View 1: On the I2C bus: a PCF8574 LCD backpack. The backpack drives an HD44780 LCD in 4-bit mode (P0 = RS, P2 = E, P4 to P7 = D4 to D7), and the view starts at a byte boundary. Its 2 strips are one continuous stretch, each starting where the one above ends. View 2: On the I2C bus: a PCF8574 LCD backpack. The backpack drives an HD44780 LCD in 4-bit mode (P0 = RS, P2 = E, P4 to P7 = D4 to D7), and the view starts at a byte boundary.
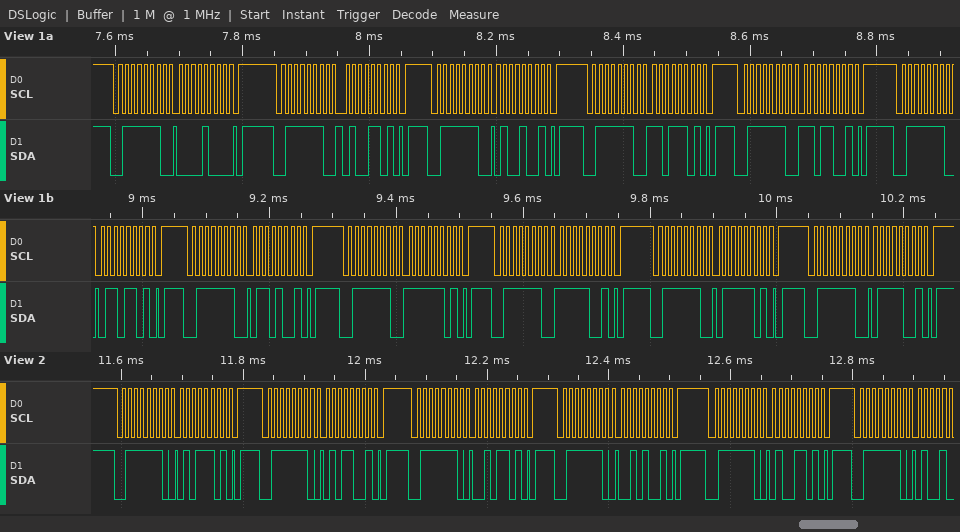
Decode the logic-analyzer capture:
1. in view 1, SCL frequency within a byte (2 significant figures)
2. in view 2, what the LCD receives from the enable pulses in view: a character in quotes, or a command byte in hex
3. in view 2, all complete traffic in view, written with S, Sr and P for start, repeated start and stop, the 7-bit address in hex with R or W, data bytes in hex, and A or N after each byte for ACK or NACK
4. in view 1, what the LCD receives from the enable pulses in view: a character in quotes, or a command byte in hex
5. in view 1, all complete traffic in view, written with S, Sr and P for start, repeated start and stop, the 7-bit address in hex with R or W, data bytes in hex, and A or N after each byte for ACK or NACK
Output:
100 kHz
'R'
S 3FW A 5D A P S 3FW A 59 A P S 3FW A 2D A P S 3FW A 29 A P S 3FW A 4D A P S 3FW A
'M' 'o'
S 3FW A 08 A P S 3FW A 4D A P S 3FW A 49 A P S 3FW A DD A P S 3FW A D9 A P S 3FW A 6D A P S 3FW A 69 A P S 3FW A FD A P S 3FW A F9 A P S 3FW A 7D A P S 3FW A 79 A P
